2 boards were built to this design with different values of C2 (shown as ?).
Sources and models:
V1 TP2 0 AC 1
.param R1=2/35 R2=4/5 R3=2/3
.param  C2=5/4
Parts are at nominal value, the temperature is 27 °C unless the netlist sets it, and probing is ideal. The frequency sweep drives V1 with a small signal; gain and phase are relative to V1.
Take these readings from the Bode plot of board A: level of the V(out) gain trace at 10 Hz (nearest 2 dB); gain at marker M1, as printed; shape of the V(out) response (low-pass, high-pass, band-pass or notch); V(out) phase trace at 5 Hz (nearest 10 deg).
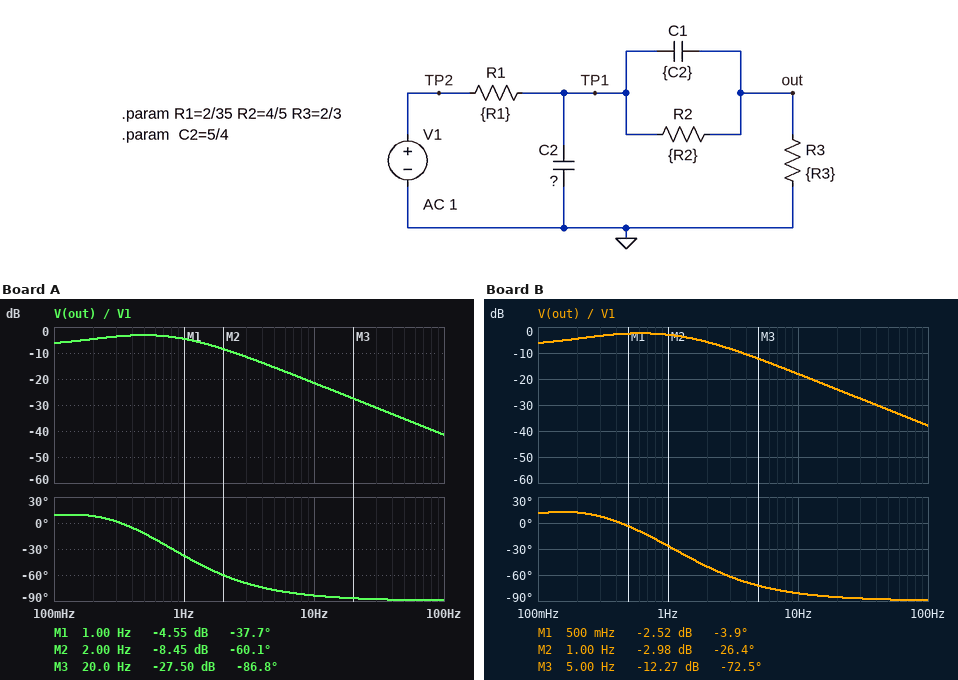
-22 dB
-4.55 dB
low-pass
-80 deg
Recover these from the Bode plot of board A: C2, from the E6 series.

3.3 F
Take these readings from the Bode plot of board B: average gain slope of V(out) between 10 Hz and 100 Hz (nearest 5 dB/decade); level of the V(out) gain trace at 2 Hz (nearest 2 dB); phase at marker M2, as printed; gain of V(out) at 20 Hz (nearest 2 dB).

-20 dB/decade
-6 dB
-26.4 deg
-24 dB
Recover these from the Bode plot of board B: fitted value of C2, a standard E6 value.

2.2 F
